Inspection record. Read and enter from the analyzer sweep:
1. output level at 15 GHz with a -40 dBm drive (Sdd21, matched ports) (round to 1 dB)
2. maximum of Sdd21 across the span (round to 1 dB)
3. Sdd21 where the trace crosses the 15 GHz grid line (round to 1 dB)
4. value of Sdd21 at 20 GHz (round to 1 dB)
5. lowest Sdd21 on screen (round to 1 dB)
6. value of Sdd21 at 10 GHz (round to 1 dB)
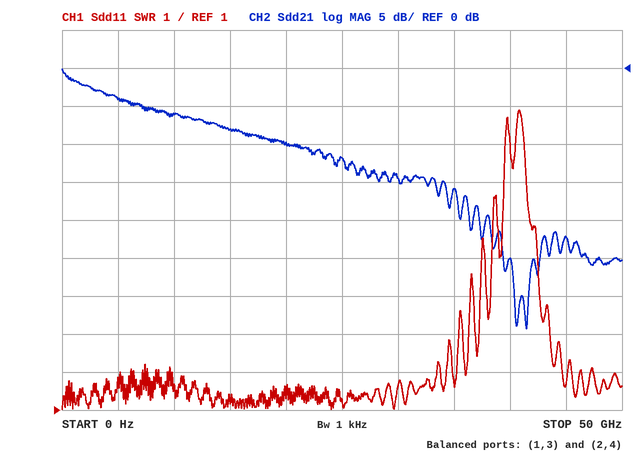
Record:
-48 dBm
0 dB
-8 dB
-10 dB
-34 dB
-6 dB
